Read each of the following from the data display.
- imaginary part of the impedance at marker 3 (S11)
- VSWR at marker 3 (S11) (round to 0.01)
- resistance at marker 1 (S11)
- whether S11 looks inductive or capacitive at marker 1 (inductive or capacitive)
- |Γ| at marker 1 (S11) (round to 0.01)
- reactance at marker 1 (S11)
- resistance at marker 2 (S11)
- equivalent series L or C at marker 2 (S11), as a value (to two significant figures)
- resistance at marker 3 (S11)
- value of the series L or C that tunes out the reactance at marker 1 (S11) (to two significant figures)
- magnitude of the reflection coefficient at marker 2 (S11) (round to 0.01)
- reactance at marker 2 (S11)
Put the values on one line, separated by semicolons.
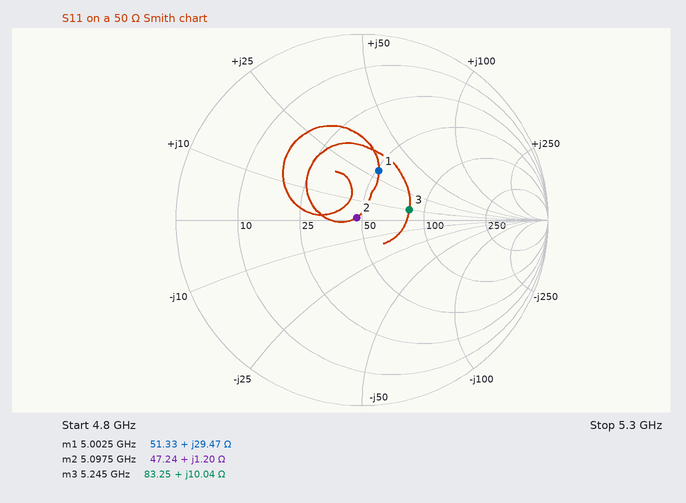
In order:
+10.04 Ω; 1.70; 51.33 Ω; inductive; 0.28; +29.47 Ω; 47.24 Ω; 37 pH; 83.25 Ω; 1.1 pF; 0.03; +1.20 Ω
